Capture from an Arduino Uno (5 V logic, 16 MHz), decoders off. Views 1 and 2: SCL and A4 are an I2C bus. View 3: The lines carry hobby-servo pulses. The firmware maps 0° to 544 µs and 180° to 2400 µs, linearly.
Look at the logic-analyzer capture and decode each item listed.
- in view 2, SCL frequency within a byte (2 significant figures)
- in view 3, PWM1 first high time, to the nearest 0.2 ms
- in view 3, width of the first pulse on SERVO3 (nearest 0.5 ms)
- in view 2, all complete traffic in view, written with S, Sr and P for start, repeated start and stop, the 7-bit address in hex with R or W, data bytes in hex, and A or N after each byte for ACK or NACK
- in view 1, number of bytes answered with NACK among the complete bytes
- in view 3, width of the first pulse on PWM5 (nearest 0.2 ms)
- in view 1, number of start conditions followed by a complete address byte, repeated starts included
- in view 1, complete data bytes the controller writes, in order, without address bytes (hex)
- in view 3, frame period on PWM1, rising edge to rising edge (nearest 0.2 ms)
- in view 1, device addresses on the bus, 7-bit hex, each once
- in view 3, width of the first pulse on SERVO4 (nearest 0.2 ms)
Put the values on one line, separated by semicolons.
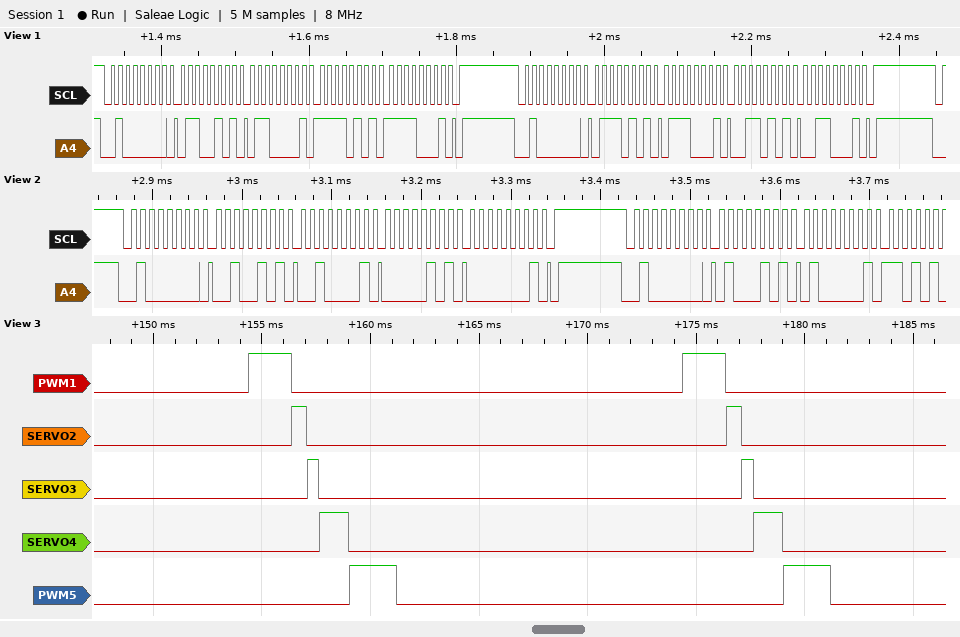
100 kHz; 2.0 ms; 0.5 ms; S 20W A 25 A 21 A 05 A 01 A P S 20W A 45 A 41 A; 0; 2.2 ms; 2; 65 61 F5 F1 75 71 35 31; 20.0 ms; 0x20; 1.4 ms
